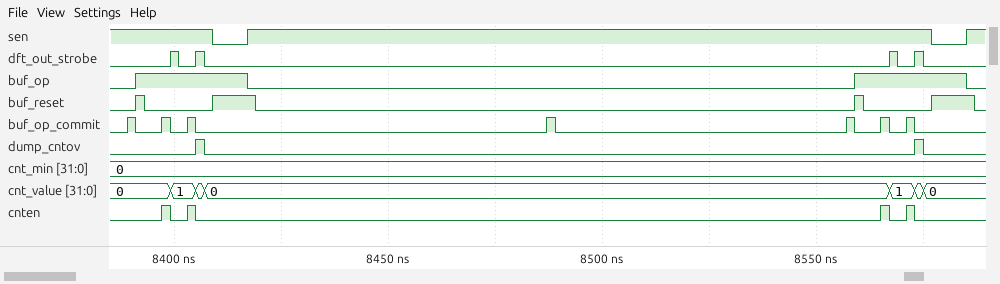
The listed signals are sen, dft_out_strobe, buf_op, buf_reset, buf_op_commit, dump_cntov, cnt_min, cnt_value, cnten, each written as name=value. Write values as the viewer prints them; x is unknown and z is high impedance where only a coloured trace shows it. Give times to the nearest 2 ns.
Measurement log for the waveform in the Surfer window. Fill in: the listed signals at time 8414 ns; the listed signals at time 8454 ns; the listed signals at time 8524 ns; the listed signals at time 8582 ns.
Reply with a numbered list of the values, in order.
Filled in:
1. sen=0, dft_out_strobe=0, buf_op=1, buf_reset=1, buf_op_commit=0, dump_cntov=0, cnt_min=0, cnt_value=0, cnten=0
2. sen=1, dft_out_strobe=0, buf_op=0, buf_reset=0, buf_op_commit=0, dump_cntov=0, cnt_min=0, cnt_value=0, cnten=0
3. sen=1, dft_out_strobe=0, buf_op=0, buf_reset=0, buf_op_commit=0, dump_cntov=0, cnt_min=0, cnt_value=0, cnten=0
4. sen=0, dft_out_strobe=0, buf_op=1, buf_reset=1, buf_op_commit=0, dump_cntov=0, cnt_min=0, cnt_value=0, cnten=0
